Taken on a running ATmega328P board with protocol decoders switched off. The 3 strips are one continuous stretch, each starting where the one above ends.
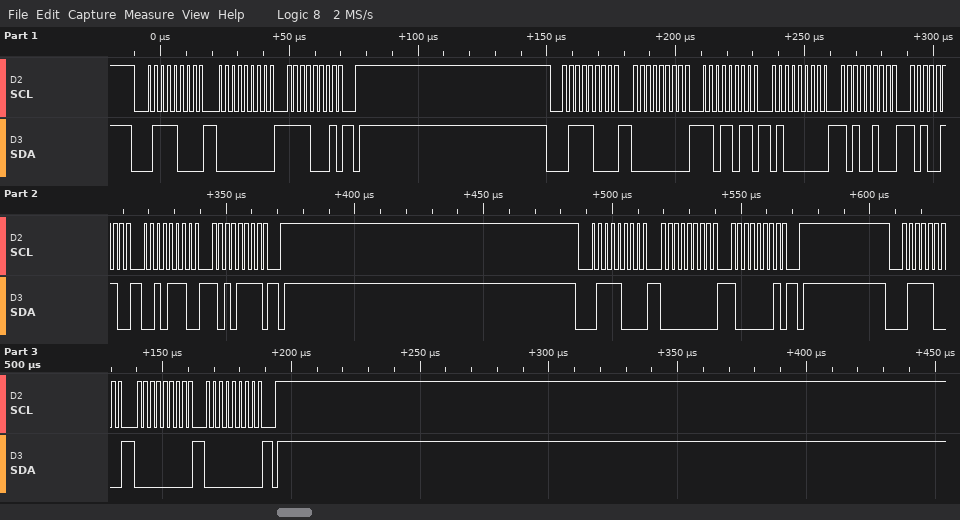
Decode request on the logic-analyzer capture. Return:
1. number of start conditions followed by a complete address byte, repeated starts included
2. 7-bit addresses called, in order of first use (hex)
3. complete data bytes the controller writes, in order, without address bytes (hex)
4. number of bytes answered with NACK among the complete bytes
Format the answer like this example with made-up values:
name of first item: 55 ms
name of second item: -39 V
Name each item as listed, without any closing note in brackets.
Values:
number of start conditions followed by a complete address byte, repeated starts included: 4
7-bit addresses called, in order of first use: 0x3C
complete data bytes the controller writes, in order, without address bytes: 00 F1 00 DB 40 A4 A6 2E AF 00 81 00 00
number of bytes answered with NACK among the complete bytes: 0
